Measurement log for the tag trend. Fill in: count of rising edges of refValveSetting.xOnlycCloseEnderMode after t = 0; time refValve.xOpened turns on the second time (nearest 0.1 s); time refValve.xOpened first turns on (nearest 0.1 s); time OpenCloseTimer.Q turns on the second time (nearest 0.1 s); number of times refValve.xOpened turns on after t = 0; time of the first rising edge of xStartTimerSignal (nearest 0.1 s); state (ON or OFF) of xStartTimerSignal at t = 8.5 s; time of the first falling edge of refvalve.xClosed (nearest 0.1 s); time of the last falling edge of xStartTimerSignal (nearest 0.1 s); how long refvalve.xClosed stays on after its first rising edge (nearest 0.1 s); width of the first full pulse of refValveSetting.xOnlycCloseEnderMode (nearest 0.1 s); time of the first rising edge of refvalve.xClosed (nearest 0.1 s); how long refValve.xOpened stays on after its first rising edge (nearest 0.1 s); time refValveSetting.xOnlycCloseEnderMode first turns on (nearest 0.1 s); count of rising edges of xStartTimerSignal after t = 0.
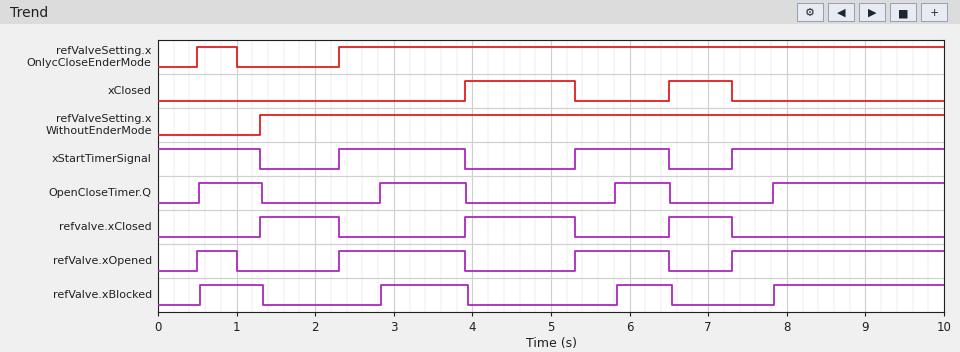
2
2.3 s
0.5 s
2.8 s
4
2.3 s
ON
2.3 s
6.5 s
1.0 s
0.5 s
1.3 s
0.5 s
0.5 s
3
